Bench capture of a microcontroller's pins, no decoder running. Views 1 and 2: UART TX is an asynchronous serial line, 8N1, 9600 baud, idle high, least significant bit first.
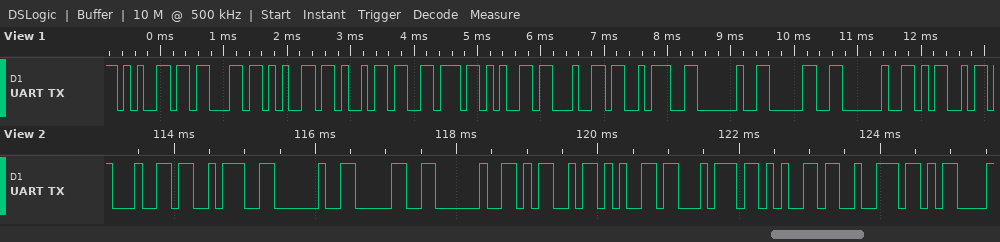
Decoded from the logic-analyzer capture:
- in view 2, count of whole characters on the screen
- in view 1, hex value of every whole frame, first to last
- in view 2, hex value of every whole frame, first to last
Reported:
11
0x65 0x63 0x65 0x69 0x76 0x65 0x64 0x3A 0x20 0x30 0x20 0x4D
64 3A 20 30 20 4D 65 74 65 72 0D
